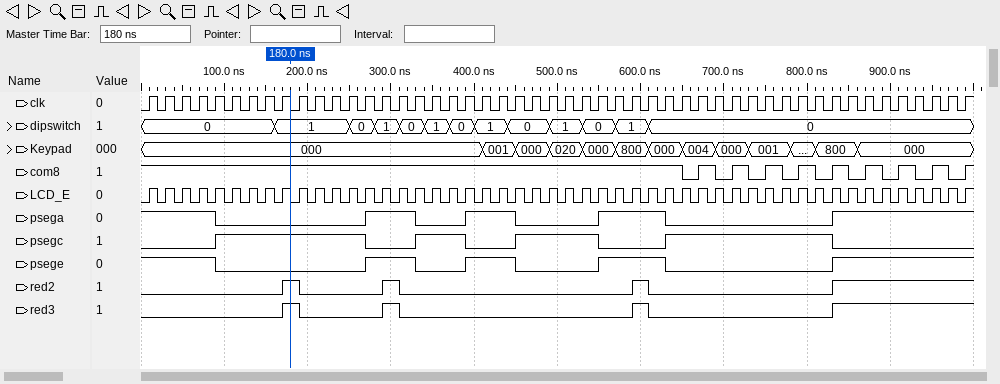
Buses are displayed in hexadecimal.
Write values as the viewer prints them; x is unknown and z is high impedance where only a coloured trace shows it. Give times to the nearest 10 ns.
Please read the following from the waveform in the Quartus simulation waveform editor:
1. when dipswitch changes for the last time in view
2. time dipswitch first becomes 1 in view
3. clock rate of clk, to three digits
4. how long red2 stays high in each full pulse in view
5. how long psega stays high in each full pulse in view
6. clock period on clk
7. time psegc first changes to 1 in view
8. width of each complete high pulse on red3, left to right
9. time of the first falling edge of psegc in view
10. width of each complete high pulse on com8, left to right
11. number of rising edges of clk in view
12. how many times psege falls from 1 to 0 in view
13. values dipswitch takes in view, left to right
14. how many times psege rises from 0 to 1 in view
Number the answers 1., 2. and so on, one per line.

1. 610 ns
2. 160 ns
3. 50.0 MHz
4. 20 ns, 20 ns, 20 ns
5. 60 ns, 60 ns, 80 ns
6. 20 ns
7. 90 ns
8. 20 ns, 20 ns, 20 ns
9. 270 ns
10. 20 ns, 20 ns, 20 ns, 20 ns, 20 ns, 20 ns, 20 ns, 20 ns
11. 50
12. 4
13. 0, 1, 0, 1, 0, 1, 0, 1, 0, 1, 0, 1, 0
14. 4
